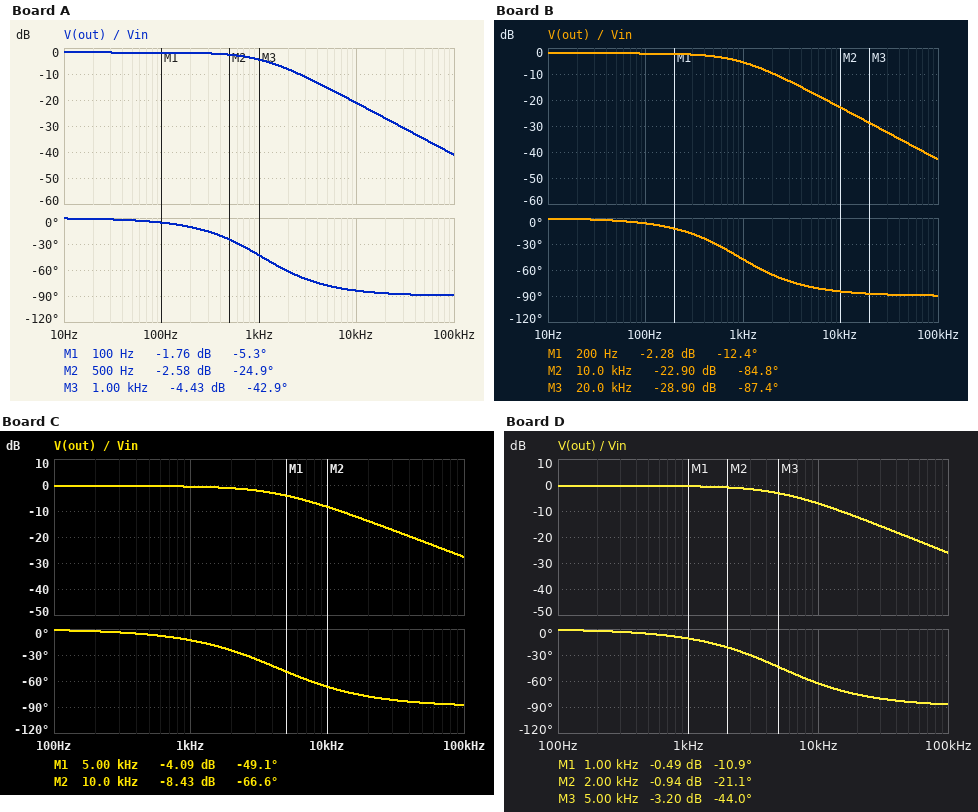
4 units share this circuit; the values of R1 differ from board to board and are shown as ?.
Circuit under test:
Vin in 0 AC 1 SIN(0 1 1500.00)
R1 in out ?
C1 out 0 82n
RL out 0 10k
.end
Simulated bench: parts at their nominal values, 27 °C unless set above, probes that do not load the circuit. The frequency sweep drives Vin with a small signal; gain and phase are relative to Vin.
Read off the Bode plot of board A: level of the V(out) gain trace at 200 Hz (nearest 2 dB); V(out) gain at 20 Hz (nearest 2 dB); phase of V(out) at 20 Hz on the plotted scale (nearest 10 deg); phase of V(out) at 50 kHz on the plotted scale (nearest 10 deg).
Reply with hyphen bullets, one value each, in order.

- -2 dB
- -2 dB
- 0 deg
- -90 deg
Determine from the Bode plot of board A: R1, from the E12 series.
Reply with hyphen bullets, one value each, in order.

- 2.2 kΩ
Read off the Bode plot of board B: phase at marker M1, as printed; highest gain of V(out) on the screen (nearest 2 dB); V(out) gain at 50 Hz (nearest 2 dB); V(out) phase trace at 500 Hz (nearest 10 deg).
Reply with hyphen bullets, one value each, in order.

- -12.4 deg
- -2 dB
- -2 dB
- -30 deg
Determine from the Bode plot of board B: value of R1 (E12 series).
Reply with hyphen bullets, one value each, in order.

- 2.7 kΩ
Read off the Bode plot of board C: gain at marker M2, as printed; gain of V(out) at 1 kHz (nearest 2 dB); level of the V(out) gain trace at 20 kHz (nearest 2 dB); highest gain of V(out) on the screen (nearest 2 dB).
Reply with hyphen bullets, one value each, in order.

- -8.43 dB
- 0 dB
- -14 dB
- 0 dB
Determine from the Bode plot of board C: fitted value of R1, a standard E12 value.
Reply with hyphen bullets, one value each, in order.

- 470 Ω
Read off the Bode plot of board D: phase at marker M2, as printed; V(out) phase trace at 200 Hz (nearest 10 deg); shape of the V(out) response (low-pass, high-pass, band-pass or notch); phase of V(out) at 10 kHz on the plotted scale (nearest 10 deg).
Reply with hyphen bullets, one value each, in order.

- -21.1 deg
- 0 deg
- low-pass
- -60 deg
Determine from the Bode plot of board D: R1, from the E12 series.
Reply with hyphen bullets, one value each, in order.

- 390 Ω
